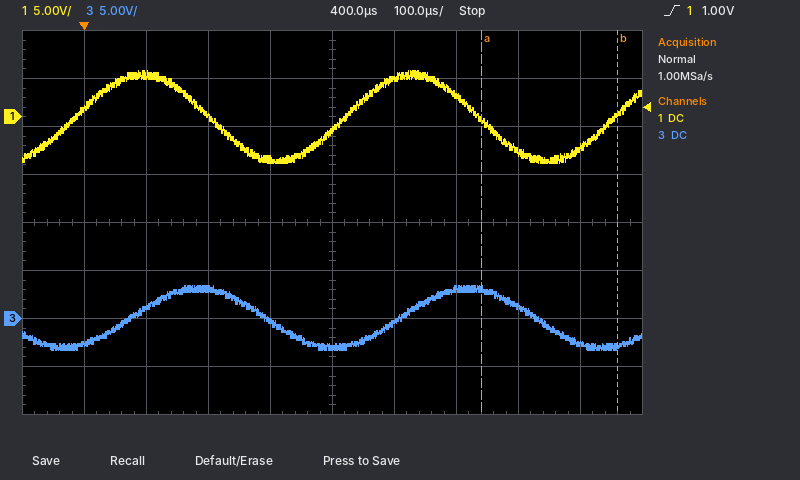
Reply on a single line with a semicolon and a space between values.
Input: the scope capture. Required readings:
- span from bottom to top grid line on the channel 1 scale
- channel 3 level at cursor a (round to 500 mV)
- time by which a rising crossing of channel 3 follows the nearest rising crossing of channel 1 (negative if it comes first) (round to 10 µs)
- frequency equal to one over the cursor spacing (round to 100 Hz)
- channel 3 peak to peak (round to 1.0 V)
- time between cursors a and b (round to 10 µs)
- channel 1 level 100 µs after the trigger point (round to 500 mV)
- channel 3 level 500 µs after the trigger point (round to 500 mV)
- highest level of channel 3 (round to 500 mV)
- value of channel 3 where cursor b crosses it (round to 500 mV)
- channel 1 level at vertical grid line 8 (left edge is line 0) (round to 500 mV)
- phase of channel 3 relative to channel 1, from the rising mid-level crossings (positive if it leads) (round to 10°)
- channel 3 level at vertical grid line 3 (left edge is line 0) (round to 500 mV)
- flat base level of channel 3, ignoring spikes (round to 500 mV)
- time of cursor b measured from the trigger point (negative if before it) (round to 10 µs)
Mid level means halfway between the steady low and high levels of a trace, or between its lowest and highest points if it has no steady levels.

40 V; 3.0 V; +90 µs; 4.5 kHz; 7.0 V; 220 µs; 4.5 V; -500 mV; 3.5 V; -3.0 V; -3.5 V; -70°; 3.0 V; -3.0 V; +860 µs
